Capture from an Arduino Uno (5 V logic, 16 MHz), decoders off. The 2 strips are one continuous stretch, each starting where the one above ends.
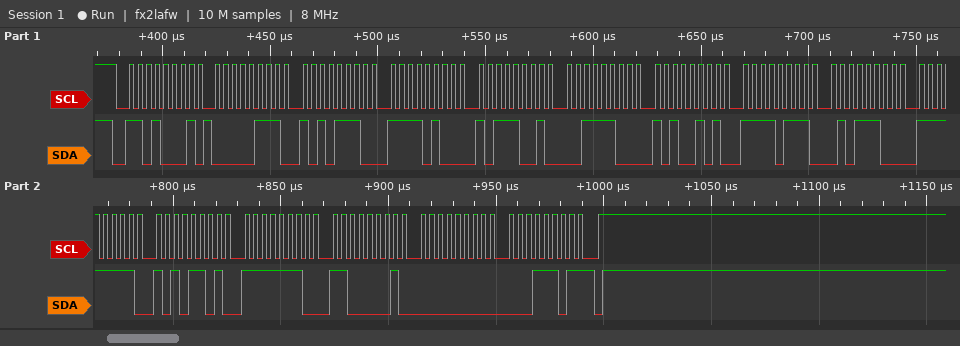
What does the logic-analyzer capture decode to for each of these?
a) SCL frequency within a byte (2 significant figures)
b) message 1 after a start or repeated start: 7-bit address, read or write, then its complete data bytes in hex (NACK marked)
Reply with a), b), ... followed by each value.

a) 250 kHz
b) 0x68 read: 07 AE F4 B9 3C A5 F7 5C FF AD FE C1 00 1D NACK
